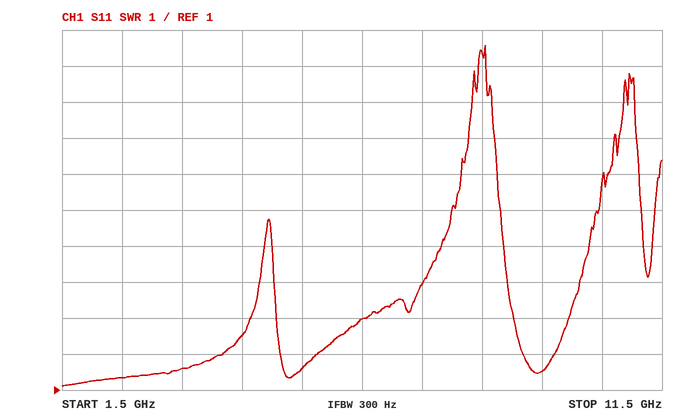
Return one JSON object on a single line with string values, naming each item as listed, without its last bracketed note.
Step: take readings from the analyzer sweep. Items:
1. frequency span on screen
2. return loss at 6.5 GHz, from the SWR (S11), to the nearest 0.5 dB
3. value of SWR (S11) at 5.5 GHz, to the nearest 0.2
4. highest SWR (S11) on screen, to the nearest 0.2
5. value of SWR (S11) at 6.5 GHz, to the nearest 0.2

{"frequency span on screen": "10 GHz", "return loss at 6.5 GHz, from the SWR (S11), to the nearest 0.5 dB": "6.0 dB", "value of SWR (S11) at 5.5 GHz, to the nearest 0.2": "1.6", "highest SWR (S11) on screen, to the nearest 0.2": "10.6", "value of SWR (S11) at 6.5 GHz, to the nearest 0.2": "3.0"}
